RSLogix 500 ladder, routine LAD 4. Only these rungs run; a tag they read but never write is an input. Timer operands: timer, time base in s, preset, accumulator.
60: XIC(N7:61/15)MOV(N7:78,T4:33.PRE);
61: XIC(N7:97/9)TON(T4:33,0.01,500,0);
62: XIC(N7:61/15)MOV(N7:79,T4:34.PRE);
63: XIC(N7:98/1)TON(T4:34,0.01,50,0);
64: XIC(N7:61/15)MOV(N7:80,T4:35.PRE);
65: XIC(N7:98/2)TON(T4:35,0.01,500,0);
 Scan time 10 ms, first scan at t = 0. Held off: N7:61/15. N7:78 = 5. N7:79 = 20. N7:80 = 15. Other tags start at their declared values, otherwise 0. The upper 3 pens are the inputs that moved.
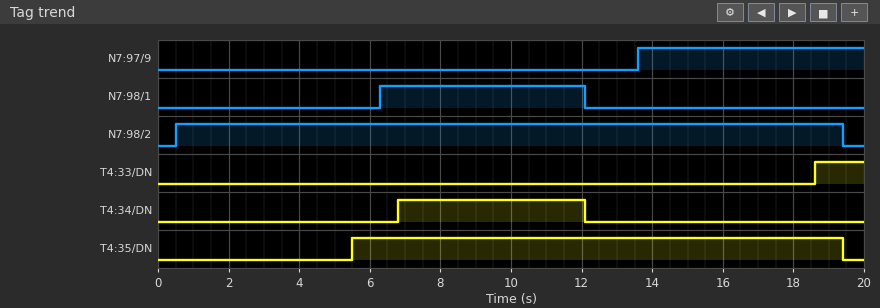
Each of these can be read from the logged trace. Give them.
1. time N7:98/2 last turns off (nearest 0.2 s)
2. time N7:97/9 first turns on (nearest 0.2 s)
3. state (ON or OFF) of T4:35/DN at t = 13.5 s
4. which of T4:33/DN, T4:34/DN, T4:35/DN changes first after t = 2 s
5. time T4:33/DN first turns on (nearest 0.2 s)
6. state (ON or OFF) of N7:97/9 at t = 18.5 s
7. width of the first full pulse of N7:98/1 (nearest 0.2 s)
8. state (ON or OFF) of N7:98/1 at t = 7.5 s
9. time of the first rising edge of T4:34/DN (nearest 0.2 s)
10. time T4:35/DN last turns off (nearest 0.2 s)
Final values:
19.4 s
13.6 s
ON
T4:35/DN
18.6 s
ON
5.8 s
ON
6.8 s
19.4 s
